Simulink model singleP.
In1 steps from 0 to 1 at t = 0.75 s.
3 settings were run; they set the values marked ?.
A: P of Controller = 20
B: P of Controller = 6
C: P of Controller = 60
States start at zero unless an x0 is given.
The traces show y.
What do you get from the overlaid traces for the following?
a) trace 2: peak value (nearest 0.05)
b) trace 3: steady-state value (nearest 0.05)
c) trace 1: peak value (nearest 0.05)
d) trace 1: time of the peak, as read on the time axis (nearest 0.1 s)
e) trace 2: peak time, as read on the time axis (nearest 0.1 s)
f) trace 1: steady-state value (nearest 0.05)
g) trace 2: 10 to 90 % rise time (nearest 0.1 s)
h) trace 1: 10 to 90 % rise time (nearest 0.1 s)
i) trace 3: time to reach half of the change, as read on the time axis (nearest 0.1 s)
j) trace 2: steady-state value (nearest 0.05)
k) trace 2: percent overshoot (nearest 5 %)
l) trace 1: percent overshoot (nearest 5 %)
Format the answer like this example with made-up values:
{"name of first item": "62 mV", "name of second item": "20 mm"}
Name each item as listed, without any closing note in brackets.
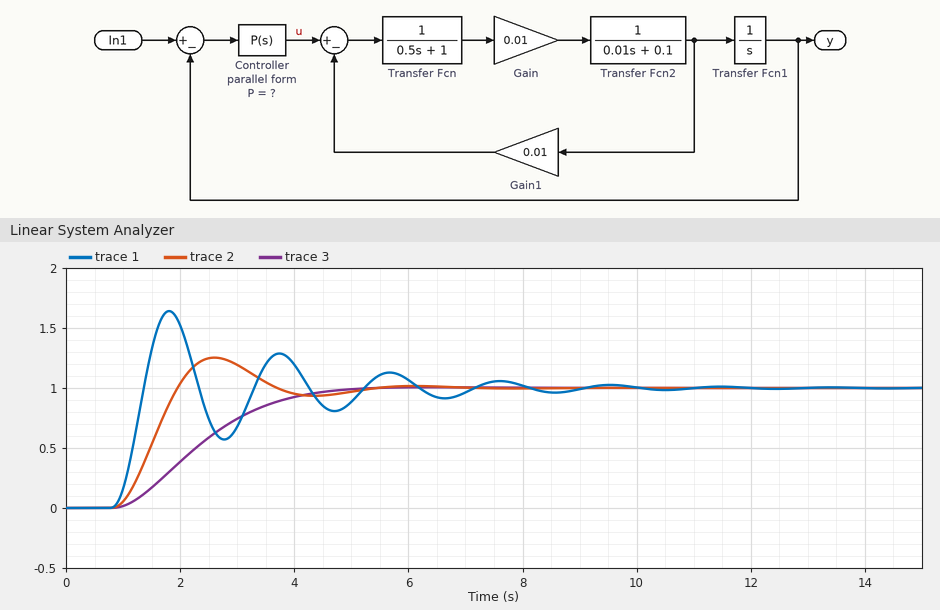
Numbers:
{"trace 2: peak value": "1.25", "trace 3: steady-state value": "1.00", "trace 1: peak value": "1.65", "trace 1: time of the peak, as read on the time axis": "1.8 s", "trace 2: peak time, as read on the time axis": "2.6 s", "trace 1: steady-state value": "1.00", "trace 2: 10 to 90 % rise time": "0.8 s", "trace 1: 10 to 90 % rise time": "0.4 s", "trace 3: time to reach half of the change, as read on the time axis": "2.3 s", "trace 2: steady-state value": "1.00", "trace 2: percent overshoot": "25 %", "trace 1: percent overshoot": "65 %"}
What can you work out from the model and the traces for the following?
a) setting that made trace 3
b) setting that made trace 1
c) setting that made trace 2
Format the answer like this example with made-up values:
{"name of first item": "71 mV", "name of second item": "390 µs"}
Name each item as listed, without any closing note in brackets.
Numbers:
{"setting that made trace 3": "B", "setting that made trace 1": "C", "setting that made trace 2": "A"}
